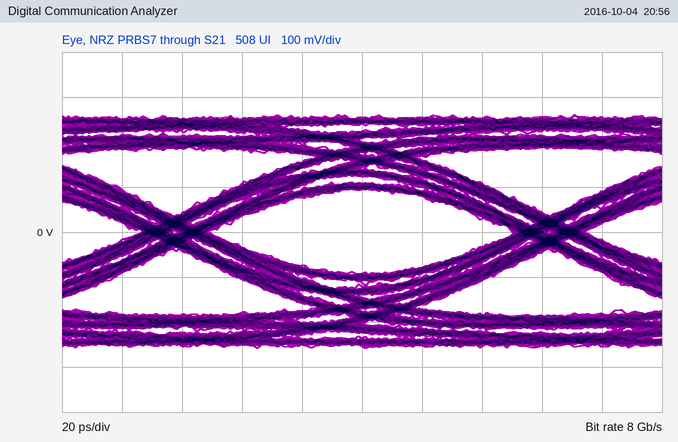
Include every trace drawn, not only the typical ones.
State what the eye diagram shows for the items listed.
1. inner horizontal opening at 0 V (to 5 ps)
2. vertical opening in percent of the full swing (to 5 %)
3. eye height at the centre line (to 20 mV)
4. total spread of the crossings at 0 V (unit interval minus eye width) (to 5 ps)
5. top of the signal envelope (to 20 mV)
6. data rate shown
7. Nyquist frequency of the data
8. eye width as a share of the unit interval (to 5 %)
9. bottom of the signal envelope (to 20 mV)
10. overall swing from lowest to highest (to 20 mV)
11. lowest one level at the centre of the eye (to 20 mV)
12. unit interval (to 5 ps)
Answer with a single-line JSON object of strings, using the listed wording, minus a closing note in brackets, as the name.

{"inner horizontal opening at 0 V": "100 ps", "vertical opening in percent of the full swing": "35 %", "eye height at the centre line": "180 mV", "total spread of the crossings at 0 V (unit interval minus eye width)": "25 ps", "top of the signal envelope": "260 mV", "data rate shown": "8 Gb/s", "Nyquist frequency of the data": "4 GHz", "eye width as a share of the unit interval": "80 %", "bottom of the signal envelope": "-260 mV", "overall swing from lowest to highest": "520 mV", "lowest one level at the centre of the eye": "100 mV", "unit interval": "125 ps"}
